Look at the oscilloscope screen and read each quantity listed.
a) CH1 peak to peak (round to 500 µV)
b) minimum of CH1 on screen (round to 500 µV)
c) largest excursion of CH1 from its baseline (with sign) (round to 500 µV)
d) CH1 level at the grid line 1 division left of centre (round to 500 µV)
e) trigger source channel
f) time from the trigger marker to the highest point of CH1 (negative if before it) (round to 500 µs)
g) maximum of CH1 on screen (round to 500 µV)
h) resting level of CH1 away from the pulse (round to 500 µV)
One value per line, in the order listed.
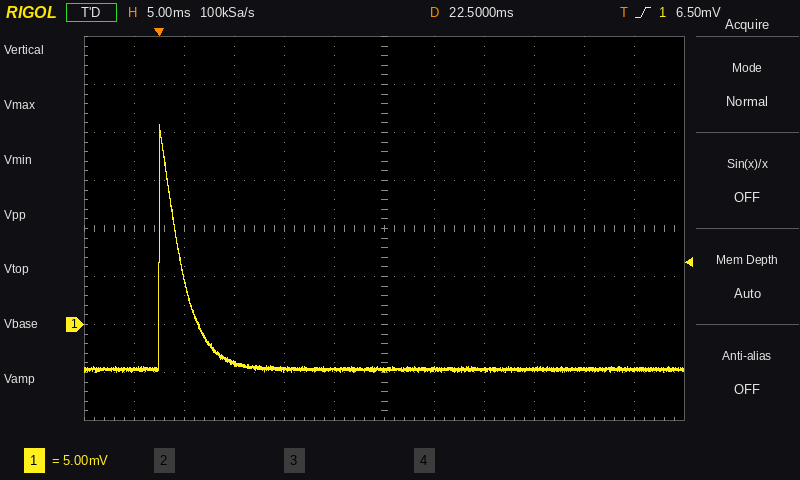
26.0 mV
-5.0 mV
+25.5 mV
-4.5 mV
CH1
0.0 ms
21.0 mV
-4.5 mV
